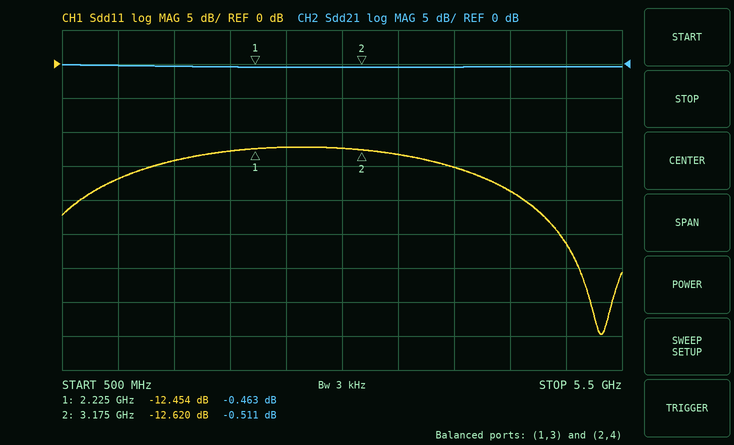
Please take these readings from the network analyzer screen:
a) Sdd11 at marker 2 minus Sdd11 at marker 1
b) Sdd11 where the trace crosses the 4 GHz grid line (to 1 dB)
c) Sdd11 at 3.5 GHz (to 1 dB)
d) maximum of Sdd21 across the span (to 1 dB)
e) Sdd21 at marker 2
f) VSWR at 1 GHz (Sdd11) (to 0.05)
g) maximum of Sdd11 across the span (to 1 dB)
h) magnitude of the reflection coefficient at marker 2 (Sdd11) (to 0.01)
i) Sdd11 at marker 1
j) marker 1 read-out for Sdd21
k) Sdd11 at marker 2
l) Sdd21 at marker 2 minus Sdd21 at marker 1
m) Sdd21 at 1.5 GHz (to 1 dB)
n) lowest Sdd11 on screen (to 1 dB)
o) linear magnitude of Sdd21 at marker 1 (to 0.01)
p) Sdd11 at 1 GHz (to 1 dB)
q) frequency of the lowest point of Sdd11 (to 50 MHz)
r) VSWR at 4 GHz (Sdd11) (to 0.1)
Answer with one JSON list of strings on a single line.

["-0.166 dB", "-15 dB", "-13 dB", "0 dB", "-0.511 dB", "1.35", "-12 dB", "0.23", "-12.454 dB", "-0.463 dB", "-12.620 dB", "-0.048 dB", "0 dB", "-40 dB", "0.95", "-17 dB", "5.30 GHz", "1.4"]
